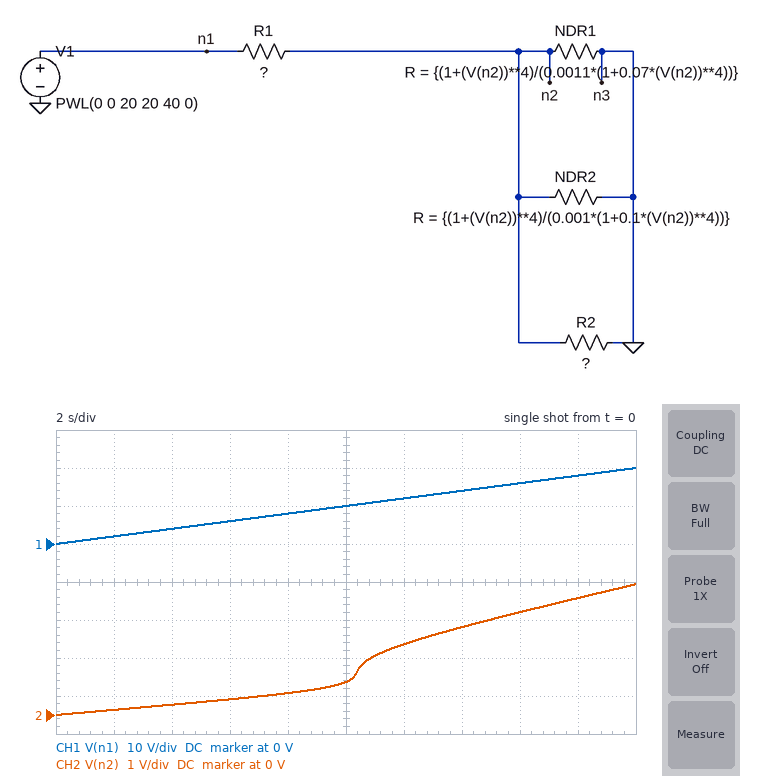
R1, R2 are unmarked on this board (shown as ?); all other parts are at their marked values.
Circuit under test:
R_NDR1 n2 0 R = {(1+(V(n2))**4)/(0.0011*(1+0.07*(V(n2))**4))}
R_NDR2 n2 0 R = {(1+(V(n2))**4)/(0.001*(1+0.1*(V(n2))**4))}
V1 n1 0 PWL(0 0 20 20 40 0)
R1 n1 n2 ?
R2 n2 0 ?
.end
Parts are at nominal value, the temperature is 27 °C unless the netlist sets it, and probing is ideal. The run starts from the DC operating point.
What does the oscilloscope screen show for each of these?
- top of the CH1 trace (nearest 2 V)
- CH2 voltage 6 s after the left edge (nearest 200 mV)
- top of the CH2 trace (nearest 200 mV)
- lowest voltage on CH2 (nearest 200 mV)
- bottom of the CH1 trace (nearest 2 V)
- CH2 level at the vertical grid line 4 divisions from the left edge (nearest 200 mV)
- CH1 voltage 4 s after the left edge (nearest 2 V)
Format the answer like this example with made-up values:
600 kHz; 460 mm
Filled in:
20 V; 400 mV; 3.4 V; 0 V; 0 V; 600 mV; 4 V
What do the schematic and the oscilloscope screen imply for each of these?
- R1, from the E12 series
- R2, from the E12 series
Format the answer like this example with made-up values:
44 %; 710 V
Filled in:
4.7 kΩ; 1.2 kΩ
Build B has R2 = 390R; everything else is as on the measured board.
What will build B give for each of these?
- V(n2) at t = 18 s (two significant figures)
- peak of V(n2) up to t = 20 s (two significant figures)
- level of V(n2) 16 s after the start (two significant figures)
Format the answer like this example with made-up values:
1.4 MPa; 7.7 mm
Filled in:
960 mV; 1.2 V; 780 mV
